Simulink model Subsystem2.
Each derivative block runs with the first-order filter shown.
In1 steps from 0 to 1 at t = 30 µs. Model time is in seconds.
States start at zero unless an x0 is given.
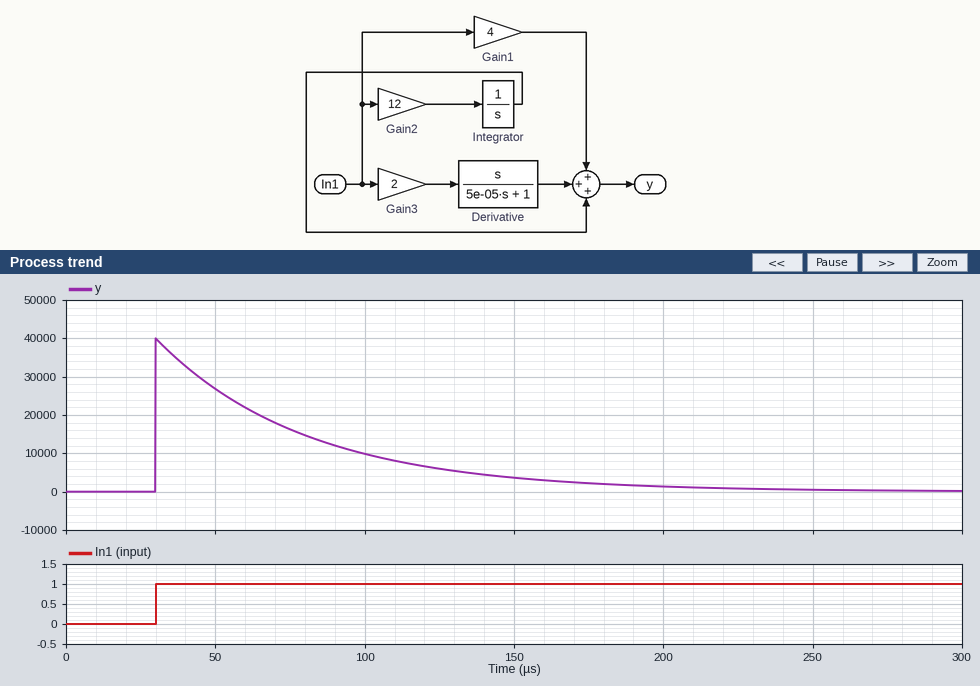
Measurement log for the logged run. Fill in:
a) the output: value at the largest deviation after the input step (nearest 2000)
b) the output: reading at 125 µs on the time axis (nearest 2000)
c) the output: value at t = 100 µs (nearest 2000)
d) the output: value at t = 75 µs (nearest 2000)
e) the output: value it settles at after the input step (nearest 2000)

40000
6000
10000
16000
0
